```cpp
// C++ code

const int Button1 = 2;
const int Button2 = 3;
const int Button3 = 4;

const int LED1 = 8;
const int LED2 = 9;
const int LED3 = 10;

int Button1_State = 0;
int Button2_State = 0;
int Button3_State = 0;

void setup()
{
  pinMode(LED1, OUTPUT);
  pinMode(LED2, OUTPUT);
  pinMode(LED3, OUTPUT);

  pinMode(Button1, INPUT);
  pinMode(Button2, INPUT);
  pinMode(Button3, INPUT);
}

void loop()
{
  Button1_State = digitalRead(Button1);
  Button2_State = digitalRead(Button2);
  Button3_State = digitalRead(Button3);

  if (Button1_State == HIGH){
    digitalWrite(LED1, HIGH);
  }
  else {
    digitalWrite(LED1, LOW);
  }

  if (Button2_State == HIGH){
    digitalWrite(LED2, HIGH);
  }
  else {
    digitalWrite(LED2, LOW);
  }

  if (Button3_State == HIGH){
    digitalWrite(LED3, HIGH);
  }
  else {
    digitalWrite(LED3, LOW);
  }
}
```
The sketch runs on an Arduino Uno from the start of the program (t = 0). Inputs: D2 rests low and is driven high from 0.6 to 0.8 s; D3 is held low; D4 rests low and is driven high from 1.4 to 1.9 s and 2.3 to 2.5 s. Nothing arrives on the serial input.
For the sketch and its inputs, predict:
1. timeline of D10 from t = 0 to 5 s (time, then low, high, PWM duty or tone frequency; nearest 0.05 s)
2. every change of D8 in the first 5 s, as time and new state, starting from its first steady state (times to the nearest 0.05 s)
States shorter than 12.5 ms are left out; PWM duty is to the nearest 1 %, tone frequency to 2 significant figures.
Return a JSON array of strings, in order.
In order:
["0 s low; 1.4 s high; 1.9 s low; 2.3 s high; 2.5 s low", "0 s low; 0.6 s high; 0.8 s low"]
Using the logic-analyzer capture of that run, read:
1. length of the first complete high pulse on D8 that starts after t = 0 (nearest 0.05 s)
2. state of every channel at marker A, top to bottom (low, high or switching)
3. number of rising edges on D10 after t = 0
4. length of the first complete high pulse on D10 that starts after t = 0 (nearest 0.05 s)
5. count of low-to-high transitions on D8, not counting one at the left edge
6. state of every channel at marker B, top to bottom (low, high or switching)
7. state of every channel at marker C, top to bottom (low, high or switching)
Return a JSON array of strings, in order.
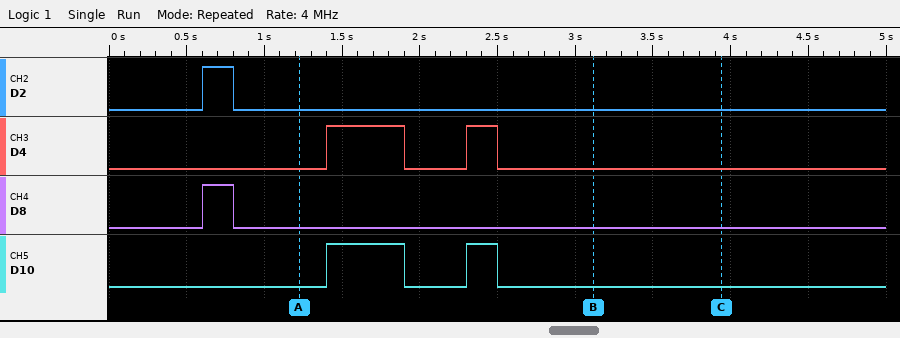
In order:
["0.20 s", "D2 low, D4 low, D8 low, D10 low", "2", "0.50 s", "1", "D2 low, D4 low, D8 low, D10 low", "D2 low, D4 low, D8 low, D10 low"]
